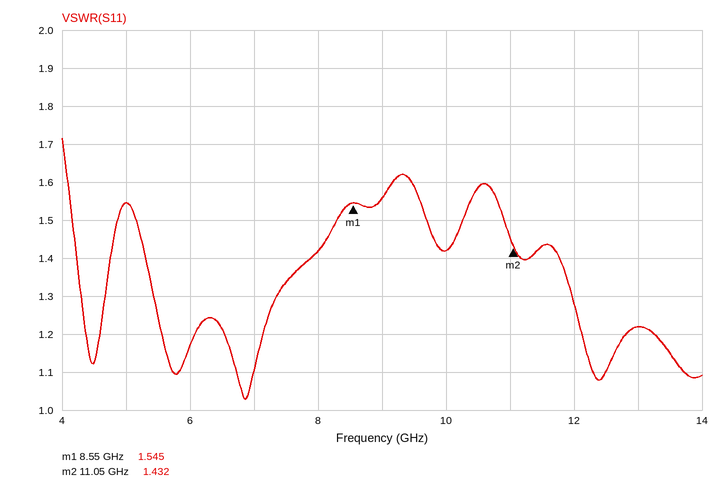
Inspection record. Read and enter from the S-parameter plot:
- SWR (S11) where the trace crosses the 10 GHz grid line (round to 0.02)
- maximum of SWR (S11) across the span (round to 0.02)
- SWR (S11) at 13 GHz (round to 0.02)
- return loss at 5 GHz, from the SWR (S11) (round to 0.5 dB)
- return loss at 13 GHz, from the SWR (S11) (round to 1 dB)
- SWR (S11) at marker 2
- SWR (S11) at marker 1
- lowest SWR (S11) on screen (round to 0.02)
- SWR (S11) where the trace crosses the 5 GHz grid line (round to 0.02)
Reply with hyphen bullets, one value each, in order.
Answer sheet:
- 1.42
- 1.72
- 1.22
- 13.5 dB
- 20 dB
- 1.432
- 1.545
- 1.02
- 1.54
